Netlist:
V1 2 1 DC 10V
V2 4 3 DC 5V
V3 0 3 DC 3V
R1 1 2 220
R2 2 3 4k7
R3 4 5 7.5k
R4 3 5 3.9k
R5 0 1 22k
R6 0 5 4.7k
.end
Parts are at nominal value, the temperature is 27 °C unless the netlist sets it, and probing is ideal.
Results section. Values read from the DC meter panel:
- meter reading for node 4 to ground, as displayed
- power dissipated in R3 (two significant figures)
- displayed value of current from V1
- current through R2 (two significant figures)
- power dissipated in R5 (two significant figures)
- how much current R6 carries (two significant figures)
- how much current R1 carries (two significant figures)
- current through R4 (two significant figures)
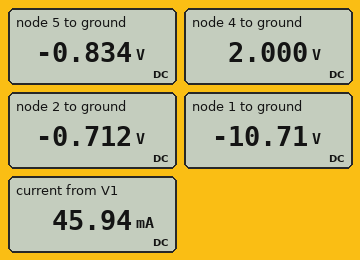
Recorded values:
2.000 V
1.1 mW
45.94 mA
490 µA
5.2 mW
180 µA
45 mA
560 µA
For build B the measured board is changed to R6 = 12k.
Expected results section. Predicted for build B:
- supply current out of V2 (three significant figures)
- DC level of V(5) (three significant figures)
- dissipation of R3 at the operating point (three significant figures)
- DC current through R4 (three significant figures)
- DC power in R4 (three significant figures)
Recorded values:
408 µA
-1.06 V
1.25 mW
497 µA
963 µW
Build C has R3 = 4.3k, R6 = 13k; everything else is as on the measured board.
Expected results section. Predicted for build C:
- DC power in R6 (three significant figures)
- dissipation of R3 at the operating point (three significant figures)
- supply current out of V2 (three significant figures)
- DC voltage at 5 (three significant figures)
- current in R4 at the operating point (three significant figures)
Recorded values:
22.2 µW
1.50 mW
590 µA
-537 mV
631 µA
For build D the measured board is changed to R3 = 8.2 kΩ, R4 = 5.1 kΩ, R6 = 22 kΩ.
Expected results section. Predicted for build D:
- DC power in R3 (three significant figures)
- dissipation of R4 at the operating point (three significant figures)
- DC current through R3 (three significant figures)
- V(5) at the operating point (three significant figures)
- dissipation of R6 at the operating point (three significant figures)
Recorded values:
1.06 mW
826 µW
359 µA
-947 mV
40.8 µW
